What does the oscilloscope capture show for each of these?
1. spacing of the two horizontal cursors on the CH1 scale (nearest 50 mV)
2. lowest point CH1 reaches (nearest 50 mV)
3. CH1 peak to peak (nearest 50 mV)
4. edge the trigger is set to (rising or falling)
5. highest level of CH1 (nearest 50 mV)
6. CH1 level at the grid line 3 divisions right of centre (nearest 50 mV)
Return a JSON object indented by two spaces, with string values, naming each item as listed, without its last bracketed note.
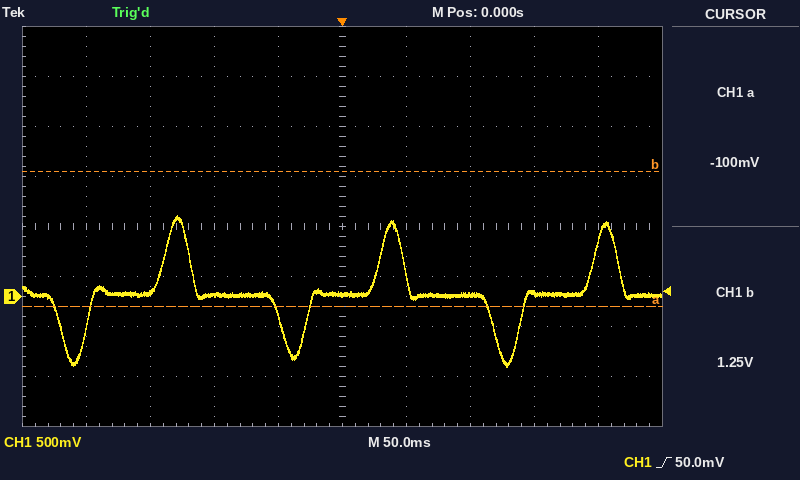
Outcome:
{
  "spacing of the two horizontal cursors on the CH1 scale": "1.35 V",
  "lowest point CH1 reaches": "-700 mV",
  "CH1 peak to peak": "1.50 V",
  "edge the trigger is set to": "rising",
  "highest level of CH1": "800 mV",
  "CH1 level at the grid line 3 divisions right of centre": "50 mV"
}
